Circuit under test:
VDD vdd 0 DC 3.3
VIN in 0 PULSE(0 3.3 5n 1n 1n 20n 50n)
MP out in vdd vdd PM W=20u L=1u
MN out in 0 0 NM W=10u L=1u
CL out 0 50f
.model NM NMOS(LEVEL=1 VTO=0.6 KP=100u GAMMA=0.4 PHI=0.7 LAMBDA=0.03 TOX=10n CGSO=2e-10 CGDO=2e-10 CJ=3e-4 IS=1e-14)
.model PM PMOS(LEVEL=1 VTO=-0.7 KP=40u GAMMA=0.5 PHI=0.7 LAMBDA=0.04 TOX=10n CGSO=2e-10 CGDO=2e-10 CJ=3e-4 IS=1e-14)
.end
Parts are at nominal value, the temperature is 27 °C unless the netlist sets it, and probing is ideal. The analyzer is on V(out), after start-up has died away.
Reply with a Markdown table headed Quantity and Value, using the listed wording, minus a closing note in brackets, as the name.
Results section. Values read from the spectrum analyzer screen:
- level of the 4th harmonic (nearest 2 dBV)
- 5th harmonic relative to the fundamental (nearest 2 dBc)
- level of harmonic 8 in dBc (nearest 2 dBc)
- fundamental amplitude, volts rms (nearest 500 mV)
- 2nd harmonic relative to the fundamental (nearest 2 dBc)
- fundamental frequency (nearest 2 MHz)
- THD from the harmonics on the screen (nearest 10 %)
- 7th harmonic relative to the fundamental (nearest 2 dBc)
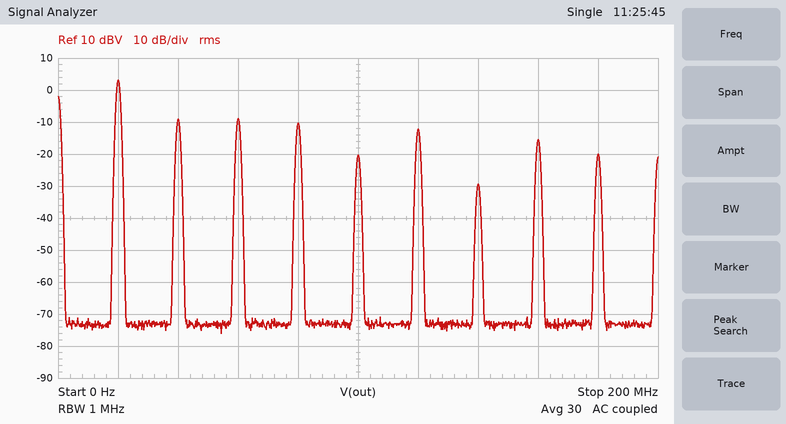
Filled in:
| Quantity | Value |
|---|---|
| level of the 4th harmonic | -10 dBV |
| 5th harmonic relative to the fundamental | -24 dBc |
| level of harmonic 8 in dBc | -18 dBc |
| fundamental amplitude, volts rms | 1.5 V |
| 2nd harmonic relative to the fundamental | -12 dBc |
| fundamental frequency | 20 MHz |
| THD from the harmonics on the screen | 50 % |
| 7th harmonic relative to the fundamental | -32 dBc |
